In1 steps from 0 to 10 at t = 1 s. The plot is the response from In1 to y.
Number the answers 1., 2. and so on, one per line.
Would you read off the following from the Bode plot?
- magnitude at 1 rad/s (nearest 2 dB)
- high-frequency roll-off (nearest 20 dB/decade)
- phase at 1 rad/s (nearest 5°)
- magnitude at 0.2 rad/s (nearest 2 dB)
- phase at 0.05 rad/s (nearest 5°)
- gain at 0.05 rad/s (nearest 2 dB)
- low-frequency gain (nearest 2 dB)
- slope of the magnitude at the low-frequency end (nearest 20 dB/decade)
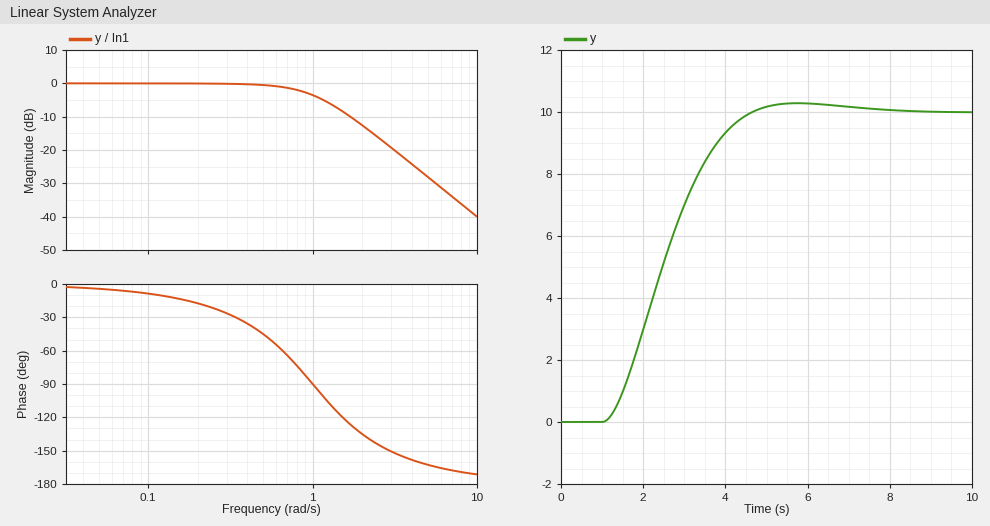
1. -4 dB
2. -40 dB/decade
3. -90°
4. 0 dB
5. -5°
6. 0 dB
7. 0 dB
8. 0 dB/decade
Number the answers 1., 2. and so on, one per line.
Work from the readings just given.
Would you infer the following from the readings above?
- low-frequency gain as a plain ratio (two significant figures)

1. 1.0
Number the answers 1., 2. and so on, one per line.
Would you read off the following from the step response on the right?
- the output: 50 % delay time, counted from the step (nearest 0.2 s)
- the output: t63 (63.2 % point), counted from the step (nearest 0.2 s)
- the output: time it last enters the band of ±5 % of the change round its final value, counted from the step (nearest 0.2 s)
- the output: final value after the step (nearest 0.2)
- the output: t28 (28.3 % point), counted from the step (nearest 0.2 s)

1. 1.4 s
2. 1.8 s
3. 3.2 s
4. 10.0
5. 1.0 s
